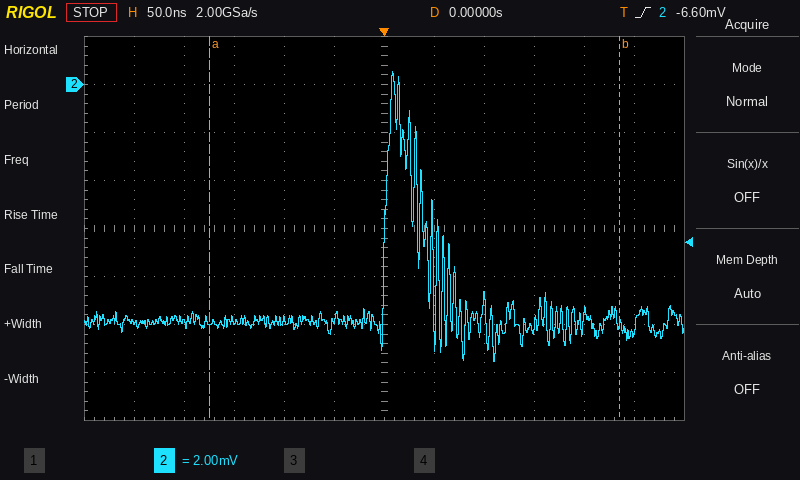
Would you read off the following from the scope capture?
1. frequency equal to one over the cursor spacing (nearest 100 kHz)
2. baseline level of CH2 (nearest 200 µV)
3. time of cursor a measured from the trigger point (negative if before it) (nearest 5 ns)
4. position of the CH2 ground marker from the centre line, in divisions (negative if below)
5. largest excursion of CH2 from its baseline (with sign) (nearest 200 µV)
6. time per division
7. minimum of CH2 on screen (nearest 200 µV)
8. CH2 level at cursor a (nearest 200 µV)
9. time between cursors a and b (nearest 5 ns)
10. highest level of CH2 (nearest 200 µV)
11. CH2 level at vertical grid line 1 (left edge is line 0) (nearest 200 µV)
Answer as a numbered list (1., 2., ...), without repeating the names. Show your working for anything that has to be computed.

1. 1 / 410 ns ≈ 2.4 MHz
2. -9.8 mV
3. -175 ns
4. +3.0 div
5. 600 µV − (-9.8 mV) = +10.4 mV
6. 50 ns
7. -11.6 mV
8. -9.8 mV
9. 410 ns
10. 600 µV
11. -10.0 mV
